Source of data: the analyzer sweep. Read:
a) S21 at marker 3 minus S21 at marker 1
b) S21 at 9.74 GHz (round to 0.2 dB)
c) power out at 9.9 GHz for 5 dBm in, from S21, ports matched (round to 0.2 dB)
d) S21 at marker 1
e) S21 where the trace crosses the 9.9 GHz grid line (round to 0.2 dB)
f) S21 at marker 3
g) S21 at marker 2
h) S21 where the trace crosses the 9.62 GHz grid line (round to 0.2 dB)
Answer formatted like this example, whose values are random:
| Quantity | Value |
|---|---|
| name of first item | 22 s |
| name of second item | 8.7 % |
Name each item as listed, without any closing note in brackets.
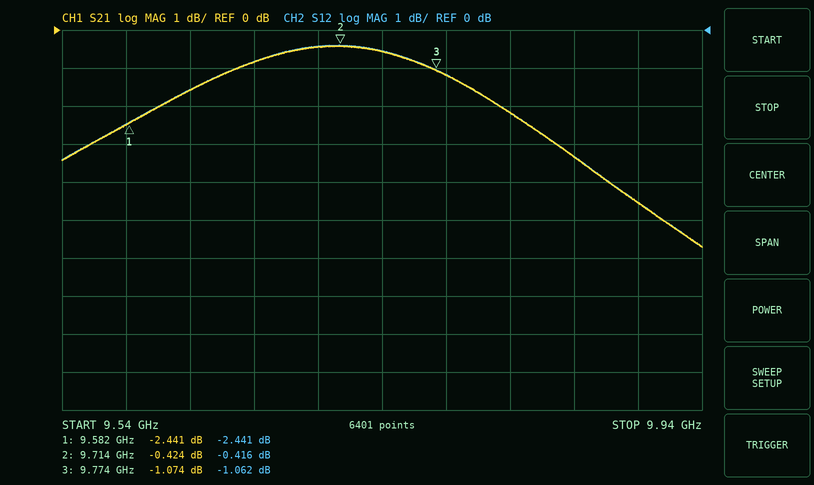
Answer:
| Quantity | Value |
|---|---|
| S21 at marker 3 minus S21 at marker 1 | 1.367 dB |
| S21 at 9.74 GHz | -0.6 dB |
| power out at 9.9 GHz for 5 dBm in, from S21, ports matched | 0.4 dBm |
| S21 at marker 1 | -2.441 dB |
| S21 where the trace crosses the 9.9 GHz grid line | -4.6 dB |
| S21 at marker 3 | -1.074 dB |
| S21 at marker 2 | -0.424 dB |
| S21 where the trace crosses the 9.62 GHz grid line | -1.6 dB |
